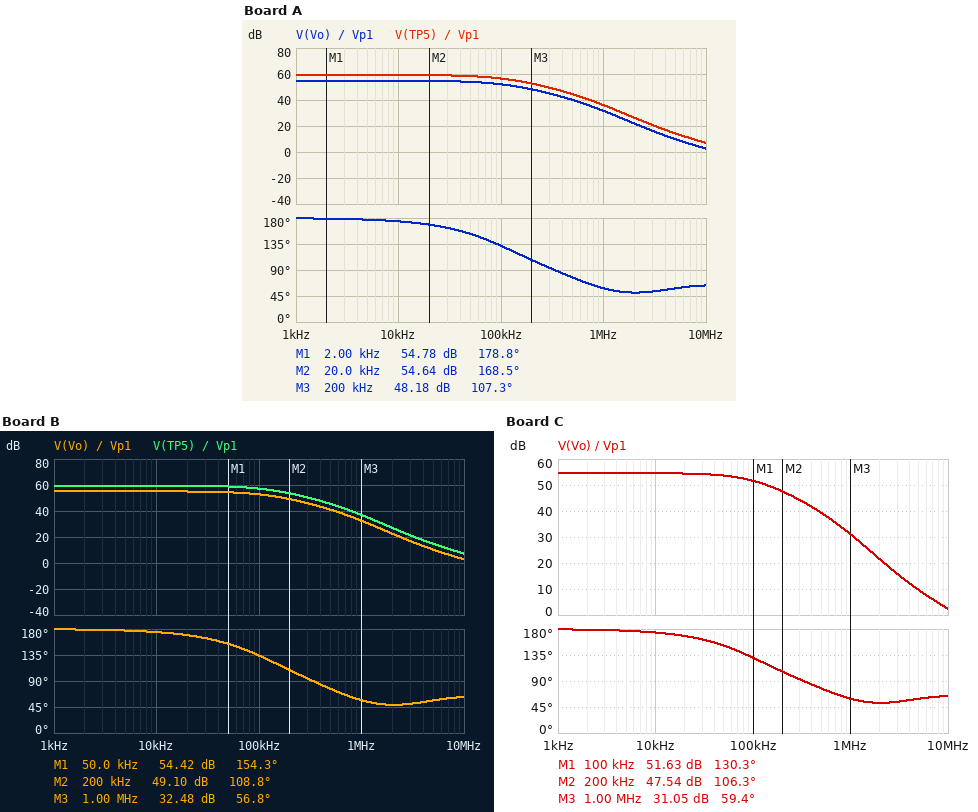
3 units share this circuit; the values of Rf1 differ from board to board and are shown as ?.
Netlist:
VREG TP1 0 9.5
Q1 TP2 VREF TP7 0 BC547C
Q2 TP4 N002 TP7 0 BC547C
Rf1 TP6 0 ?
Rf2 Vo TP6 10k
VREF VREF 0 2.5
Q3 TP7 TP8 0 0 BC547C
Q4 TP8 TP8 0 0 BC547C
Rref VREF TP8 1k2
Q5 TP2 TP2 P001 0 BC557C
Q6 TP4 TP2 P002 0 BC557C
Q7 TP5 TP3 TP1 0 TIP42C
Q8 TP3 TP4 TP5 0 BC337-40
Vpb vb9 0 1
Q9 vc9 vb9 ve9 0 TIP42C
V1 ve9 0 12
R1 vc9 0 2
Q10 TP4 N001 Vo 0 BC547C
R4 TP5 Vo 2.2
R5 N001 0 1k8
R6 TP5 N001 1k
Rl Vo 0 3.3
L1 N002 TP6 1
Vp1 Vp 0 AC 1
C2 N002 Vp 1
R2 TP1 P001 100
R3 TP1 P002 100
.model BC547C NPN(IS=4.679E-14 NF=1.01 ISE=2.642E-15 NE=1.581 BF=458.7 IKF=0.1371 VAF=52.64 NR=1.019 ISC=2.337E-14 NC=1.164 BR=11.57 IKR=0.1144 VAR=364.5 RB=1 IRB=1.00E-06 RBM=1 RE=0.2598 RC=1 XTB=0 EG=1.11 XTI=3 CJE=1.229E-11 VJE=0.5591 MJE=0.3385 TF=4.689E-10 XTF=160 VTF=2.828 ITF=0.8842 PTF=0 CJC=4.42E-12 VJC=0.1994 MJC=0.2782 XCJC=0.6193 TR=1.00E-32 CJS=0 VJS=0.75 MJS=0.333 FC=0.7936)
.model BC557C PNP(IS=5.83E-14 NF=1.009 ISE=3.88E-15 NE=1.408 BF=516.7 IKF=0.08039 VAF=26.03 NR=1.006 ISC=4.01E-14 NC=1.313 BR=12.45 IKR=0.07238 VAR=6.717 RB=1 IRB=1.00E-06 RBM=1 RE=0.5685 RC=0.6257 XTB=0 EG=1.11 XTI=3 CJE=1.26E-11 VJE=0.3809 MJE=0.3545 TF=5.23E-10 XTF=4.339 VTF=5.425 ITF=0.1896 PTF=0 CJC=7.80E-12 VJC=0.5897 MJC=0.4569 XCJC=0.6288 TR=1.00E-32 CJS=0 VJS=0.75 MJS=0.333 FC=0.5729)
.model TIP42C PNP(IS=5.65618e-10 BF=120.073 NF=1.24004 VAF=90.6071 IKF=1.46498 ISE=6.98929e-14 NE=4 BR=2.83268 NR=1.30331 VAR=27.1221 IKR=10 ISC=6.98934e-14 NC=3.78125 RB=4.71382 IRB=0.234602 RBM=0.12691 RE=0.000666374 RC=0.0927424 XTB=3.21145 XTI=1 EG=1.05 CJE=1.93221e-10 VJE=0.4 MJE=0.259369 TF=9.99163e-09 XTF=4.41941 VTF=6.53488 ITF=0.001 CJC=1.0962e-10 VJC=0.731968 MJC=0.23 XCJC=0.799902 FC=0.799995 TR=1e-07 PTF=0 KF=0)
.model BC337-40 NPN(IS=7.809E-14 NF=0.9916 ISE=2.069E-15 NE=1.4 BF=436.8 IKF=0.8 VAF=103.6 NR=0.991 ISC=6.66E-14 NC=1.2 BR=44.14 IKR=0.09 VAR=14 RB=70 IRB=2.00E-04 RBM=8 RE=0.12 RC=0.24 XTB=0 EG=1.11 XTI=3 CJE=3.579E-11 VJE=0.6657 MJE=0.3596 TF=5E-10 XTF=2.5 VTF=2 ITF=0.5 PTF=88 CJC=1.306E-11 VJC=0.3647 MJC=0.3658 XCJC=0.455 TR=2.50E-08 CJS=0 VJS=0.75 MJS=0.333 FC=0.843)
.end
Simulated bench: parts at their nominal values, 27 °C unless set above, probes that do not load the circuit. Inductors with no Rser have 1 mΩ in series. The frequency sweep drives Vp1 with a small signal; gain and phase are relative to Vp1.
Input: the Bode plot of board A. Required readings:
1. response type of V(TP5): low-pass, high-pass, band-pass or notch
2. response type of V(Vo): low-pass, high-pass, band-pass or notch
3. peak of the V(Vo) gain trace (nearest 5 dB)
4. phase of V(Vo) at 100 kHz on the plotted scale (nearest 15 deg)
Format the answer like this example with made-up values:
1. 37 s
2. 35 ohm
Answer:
1. low-pass
2. low-pass
3. 55 dB
4. 135 deg
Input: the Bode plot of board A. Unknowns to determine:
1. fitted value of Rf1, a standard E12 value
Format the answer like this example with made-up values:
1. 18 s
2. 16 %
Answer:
1. 18 kΩ
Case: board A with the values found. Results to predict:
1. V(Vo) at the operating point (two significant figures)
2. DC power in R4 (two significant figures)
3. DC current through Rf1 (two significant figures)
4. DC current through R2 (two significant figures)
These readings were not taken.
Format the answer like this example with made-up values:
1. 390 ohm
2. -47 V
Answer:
1. 3.9 V
2. 3.1 W
3. 140 µA
4. 810 µA
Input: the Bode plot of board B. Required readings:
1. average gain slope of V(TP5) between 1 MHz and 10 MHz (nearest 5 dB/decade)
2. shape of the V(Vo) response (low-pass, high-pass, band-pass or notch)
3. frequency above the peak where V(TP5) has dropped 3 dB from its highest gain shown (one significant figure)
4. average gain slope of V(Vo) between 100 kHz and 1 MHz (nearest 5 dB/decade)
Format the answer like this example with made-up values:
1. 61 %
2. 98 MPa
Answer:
1. -30 dB/decade
2. low-pass
3. 100 kHz
4. -20 dB/decade
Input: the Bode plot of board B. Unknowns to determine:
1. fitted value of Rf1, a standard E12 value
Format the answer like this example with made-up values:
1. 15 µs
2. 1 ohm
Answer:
1. 27 kΩ
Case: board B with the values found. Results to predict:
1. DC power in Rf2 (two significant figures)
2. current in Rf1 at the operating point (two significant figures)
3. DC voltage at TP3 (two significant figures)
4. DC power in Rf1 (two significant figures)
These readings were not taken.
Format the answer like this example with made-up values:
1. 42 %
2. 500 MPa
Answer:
1. 89 µW
2. 93 µA
3. 8.7 V
4. 230 µW
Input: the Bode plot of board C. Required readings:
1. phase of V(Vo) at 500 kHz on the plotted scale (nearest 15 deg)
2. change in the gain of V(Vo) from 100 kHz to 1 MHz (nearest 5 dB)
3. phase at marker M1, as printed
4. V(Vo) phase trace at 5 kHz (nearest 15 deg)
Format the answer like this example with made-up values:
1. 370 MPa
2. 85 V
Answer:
1. 75 deg
2. -20 dB
3. 130.3 deg
4. 180 deg
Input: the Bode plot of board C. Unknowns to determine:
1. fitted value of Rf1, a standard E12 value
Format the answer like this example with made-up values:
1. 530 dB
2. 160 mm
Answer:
1. 15 kΩ
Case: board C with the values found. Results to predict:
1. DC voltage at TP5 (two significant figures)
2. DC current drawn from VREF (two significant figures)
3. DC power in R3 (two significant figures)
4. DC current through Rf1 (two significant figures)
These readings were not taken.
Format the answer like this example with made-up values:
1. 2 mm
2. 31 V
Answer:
1. 7.0 V
2. 1.6 mA
3. 67 µW
4. 170 µA
